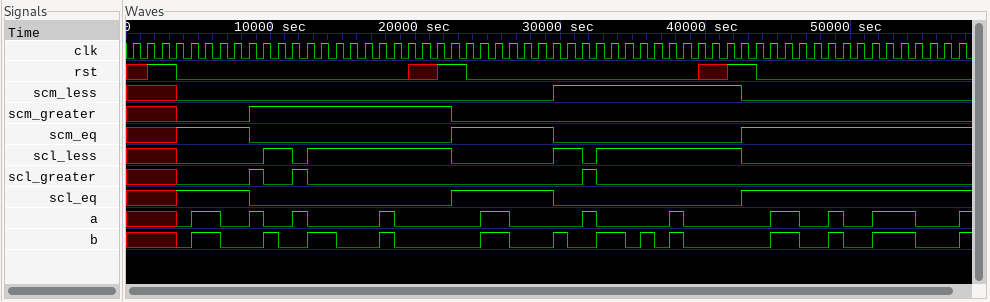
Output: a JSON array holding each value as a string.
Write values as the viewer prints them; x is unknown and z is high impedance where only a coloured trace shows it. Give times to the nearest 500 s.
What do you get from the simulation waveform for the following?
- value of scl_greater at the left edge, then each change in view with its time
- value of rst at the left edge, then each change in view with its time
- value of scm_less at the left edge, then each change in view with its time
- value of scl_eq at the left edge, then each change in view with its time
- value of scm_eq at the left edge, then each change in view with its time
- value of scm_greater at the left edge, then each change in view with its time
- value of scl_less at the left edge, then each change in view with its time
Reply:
["x, 0 at 3500 s, 1 at 8500 s, 0 at 9500 s, 1 at 11500 s, 0 at 12500 s, 1 at 31500 s, 0 at 32500 s", "x, 1 at 1500 s, 0 at 3500 s, x at 19500 s, 1 at 21500 s, 0 at 23500 s, x at 39500 s, 1 at 41500 s, 0 at 43500 s", "x, 0 at 3500 s, 1 at 29500 s, 0 at 42500 s", "x, 1 at 3500 s, 0 at 8500 s, 1 at 22500 s, 0 at 29500 s, 1 at 42500 s", "x, 1 at 3500 s, 0 at 8500 s, 1 at 22500 s, 0 at 29500 s, 1 at 42500 s", "x, 0 at 3500 s, 1 at 8500 s, 0 at 22500 s", "x, 0 at 3500 s, 1 at 9500 s, 0 at 11500 s, 1 at 12500 s, 0 at 22500 s, 1 at 29500 s, 0 at 31500 s, 1 at 32500 s, 0 at 42500 s"]
